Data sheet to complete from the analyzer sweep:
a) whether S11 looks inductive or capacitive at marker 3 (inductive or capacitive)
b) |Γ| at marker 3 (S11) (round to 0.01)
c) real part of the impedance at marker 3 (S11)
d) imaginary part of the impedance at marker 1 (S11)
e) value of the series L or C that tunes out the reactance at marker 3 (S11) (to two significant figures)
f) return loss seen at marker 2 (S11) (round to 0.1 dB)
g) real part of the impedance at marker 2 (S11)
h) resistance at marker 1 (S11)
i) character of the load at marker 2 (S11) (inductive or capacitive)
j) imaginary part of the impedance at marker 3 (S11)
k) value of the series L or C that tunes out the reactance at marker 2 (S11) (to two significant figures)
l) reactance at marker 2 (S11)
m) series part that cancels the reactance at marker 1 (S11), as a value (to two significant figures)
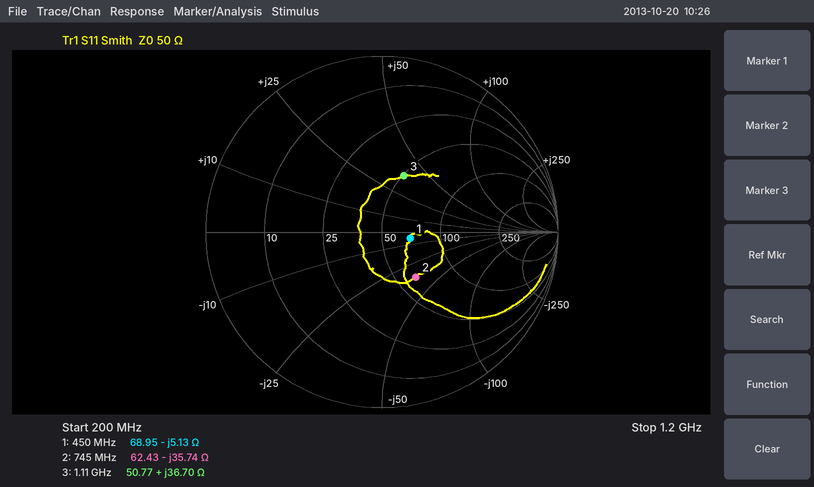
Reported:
inductive
0.34
50.77 Ω
-5.13 Ω
3.9 pF
9.9 dB
62.43 Ω
68.95 Ω
capacitive
+36.70 Ω
7.6 nH
-35.74 Ω
1.8 nH
